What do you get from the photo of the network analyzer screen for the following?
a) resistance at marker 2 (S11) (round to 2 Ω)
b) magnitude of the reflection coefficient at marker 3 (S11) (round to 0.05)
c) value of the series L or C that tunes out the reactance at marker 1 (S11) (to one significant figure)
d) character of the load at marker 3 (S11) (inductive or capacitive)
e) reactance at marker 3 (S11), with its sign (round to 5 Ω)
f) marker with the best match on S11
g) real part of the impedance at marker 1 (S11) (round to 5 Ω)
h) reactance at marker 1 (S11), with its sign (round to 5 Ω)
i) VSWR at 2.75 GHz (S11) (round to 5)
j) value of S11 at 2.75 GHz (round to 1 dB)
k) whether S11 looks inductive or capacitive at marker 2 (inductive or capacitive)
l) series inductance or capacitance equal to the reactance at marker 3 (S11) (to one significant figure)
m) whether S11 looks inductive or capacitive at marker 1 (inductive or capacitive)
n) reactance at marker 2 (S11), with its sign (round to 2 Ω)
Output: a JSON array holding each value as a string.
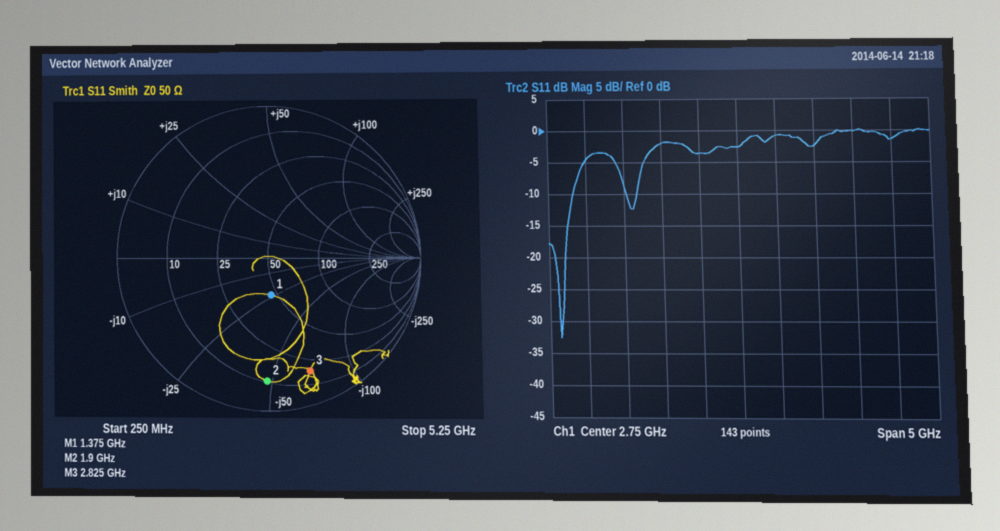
["10 Ω", "0.80", "3 nH", "capacitive", "-70 Ω", "marker 1", "45 Ω", "-25 Ω", "5", "-3 dB", "capacitive", "800 fF", "capacitive", "-48 Ω"]
